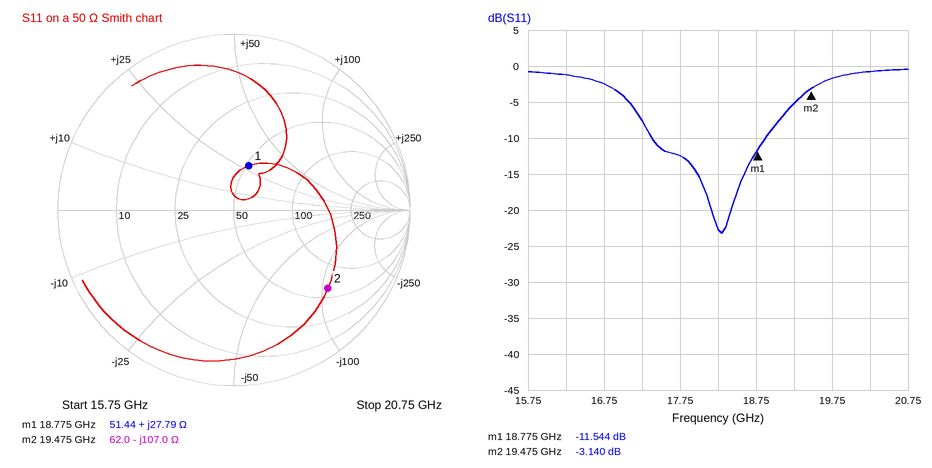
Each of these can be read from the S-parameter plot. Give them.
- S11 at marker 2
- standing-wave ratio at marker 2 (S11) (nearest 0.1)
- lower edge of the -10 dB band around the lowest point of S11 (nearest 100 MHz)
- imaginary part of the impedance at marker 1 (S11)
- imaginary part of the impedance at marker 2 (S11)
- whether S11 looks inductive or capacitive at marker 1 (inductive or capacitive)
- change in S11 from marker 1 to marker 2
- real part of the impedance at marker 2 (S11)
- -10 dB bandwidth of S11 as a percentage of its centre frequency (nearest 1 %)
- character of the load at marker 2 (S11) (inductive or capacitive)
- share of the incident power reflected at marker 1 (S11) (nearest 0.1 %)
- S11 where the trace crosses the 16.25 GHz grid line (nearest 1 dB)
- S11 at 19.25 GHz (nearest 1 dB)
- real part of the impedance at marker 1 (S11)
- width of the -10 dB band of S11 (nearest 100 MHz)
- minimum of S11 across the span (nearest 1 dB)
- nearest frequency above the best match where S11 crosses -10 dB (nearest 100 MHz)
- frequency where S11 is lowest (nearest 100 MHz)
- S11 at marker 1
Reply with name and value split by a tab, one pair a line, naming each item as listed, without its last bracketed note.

S11 at marker 2	-3.140 dB
standing-wave ratio at marker 2 (S11)	5.6
lower edge of the -10 dB band around the lowest point of S11	17.4 GHz
imaginary part of the impedance at marker 1	+27.79 Ω
imaginary part of the impedance at marker 2	-107.0 Ω
whether S11 looks inductive or capacitive at marker 1	inductive
change in S11 from marker 1 to marker 2	8.404 dB
real part of the impedance at marker 2	62.0 Ω
-10 dB bandwidth of S11 as a percentage of its centre frequency	8 %
character of the load at marker 2 (S11)	capacitive
share of the incident power reflected at marker 1 (S11)	7.0 %
S11 where the trace crosses the 16.25 GHz grid line	-1 dB
S11 at 19.25 GHz	-5 dB
real part of the impedance at marker 1	51.44 Ω
width of the -10 dB band of S11	1.5 GHz
minimum of S11 across the span	-23 dB
nearest frequency above the best match where S11 crosses -10 dB	18.9 GHz
frequency where S11 is lowest	18.3 GHz
S11 at marker 1	-11.544 dB
